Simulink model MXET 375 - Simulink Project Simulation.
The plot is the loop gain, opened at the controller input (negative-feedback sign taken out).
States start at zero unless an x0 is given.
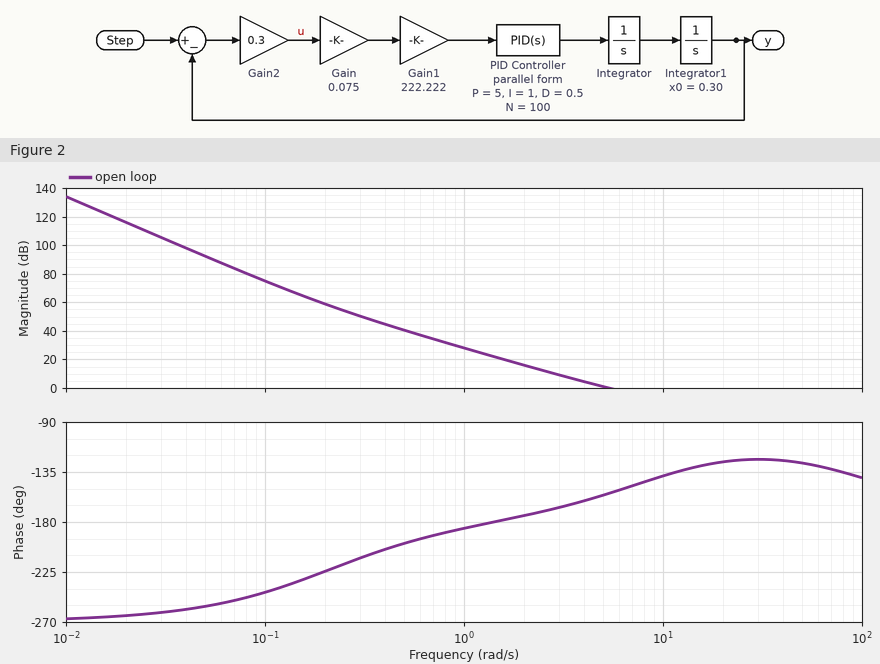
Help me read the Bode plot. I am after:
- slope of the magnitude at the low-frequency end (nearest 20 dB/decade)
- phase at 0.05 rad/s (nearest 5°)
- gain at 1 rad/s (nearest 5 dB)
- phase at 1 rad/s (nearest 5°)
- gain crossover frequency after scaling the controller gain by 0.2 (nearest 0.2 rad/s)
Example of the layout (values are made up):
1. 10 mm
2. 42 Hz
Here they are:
1. -60 dB/decade
2. -255°
3. 30 dB
4. -185°
5. 2.2 rad/s
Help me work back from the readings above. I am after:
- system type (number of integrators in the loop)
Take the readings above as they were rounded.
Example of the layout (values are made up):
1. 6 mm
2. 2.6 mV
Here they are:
1. 3
